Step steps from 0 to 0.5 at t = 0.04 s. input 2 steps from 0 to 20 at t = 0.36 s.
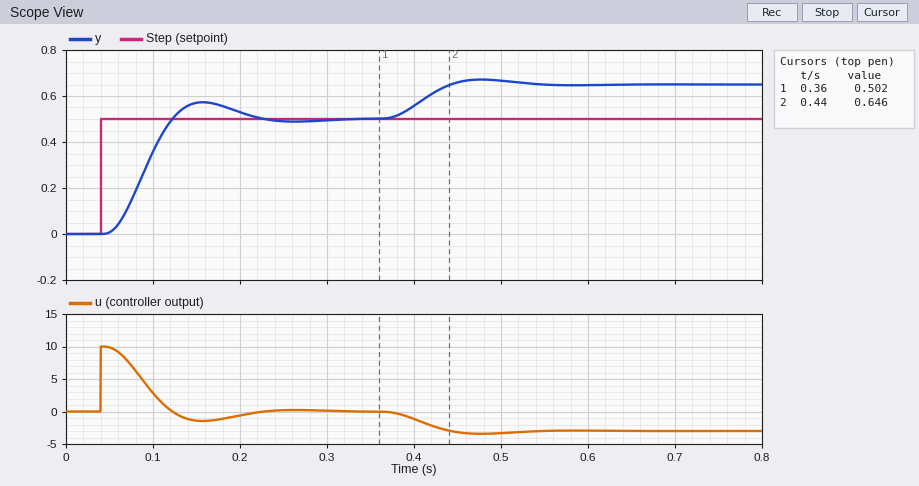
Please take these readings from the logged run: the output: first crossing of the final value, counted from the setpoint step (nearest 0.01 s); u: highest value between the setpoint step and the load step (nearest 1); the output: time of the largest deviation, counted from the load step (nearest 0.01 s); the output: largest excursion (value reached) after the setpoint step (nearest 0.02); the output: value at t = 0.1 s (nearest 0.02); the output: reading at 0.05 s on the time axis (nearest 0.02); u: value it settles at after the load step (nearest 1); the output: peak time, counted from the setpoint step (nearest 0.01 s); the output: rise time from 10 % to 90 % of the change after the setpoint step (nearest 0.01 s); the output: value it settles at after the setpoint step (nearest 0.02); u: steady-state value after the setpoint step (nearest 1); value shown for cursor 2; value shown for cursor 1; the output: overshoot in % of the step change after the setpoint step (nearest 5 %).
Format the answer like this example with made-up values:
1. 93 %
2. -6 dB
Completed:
1. 0.08 s
2. 10
3. 0.12 s
4. 0.58
5. 0.36
6. 0.00
7. -3
8. 0.12 s
9. 0.05 s
10. 0.50
11. 0
12. 0.646
13. 0.502
14. 15 %
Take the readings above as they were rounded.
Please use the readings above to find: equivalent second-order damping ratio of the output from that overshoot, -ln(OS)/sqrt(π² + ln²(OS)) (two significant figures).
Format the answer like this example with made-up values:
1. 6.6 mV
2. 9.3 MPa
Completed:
1. 0.52
